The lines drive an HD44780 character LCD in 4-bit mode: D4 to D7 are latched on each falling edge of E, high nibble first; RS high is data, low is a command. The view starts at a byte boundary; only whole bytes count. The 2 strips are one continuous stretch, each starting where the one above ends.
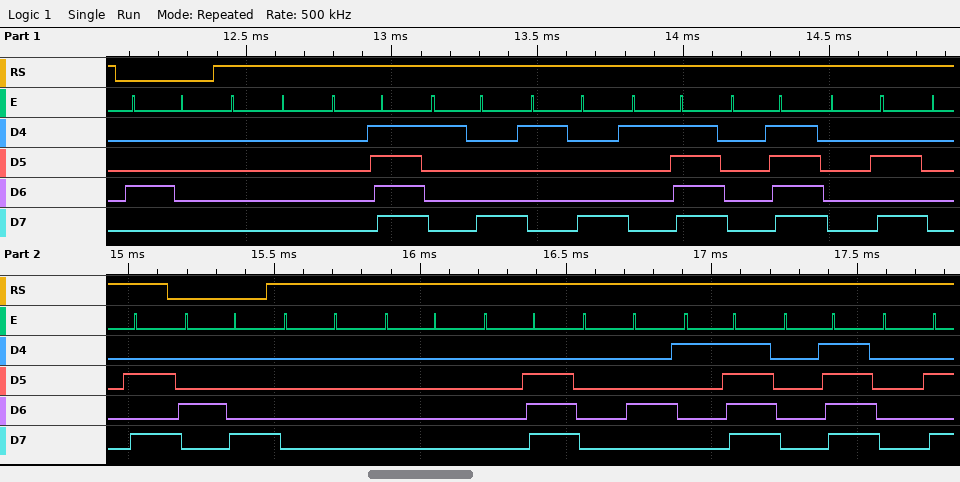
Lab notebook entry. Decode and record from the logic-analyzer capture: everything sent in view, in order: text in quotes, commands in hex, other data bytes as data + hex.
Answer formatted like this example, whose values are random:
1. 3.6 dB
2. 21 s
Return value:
1. 0x40 data 00 0F 18 18 1F 0F 0A 0A 0x48 data 00 00 0E 04 1F 0F 0A
